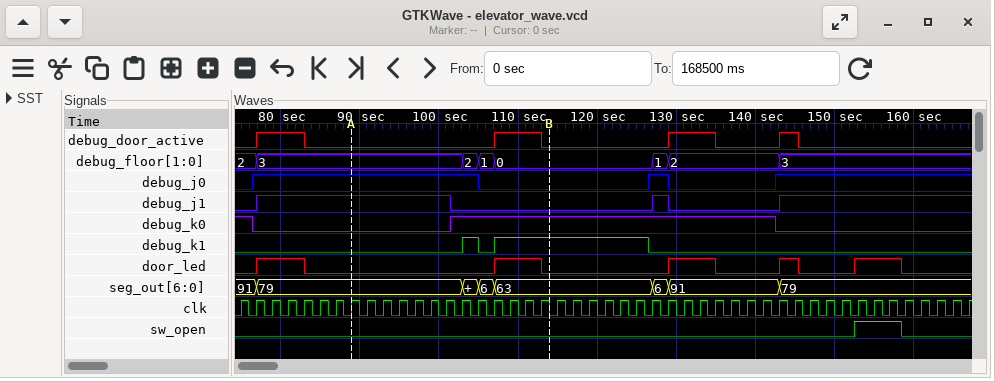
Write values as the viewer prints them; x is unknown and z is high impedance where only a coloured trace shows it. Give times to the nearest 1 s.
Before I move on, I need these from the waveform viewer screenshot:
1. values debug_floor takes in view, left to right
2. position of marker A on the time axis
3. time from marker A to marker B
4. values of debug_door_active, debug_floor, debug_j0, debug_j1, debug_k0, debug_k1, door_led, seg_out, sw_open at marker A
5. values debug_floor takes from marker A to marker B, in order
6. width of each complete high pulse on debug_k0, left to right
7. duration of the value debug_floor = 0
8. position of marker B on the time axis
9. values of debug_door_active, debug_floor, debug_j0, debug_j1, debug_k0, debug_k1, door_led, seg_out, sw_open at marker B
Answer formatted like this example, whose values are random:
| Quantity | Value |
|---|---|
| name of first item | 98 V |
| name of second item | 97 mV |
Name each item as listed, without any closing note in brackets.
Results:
| Quantity | Value |
|---|---|
| values debug_floor takes in view, left to right | 2, 3, 2, 1, 0, 1, 2, 3 |
| position of marker A on the time axis | 89 s |
| time from marker A to marker B | 25 s |
| values of debug_door_active, debug_floor, debug_j0, debug_j1, debug_k0, debug_k1, door_led, seg_out, sw_open at marker A | debug_door_active=0, debug_floor=3, debug_j0=1, debug_j1=1, debug_k0=0, debug_k1=0, door_led=0, seg_out=79, sw_open=0 |
| values debug_floor takes from marker A to marker B, in order | 3, 2, 1, 0 |
| width of each complete high pulse on debug_k0, left to right | 41 s |
| duration of the value debug_floor = 0 | 20 s |
| position of marker B on the time axis | 114 s |
| values of debug_door_active, debug_floor, debug_j0, debug_j1, debug_k0, debug_k1, door_led, seg_out, sw_open at marker B | debug_door_active=0, debug_floor=0, debug_j0=0, debug_j1=0, debug_k0=1, debug_k1=1, door_led=0, seg_out=63, sw_open=0 |
